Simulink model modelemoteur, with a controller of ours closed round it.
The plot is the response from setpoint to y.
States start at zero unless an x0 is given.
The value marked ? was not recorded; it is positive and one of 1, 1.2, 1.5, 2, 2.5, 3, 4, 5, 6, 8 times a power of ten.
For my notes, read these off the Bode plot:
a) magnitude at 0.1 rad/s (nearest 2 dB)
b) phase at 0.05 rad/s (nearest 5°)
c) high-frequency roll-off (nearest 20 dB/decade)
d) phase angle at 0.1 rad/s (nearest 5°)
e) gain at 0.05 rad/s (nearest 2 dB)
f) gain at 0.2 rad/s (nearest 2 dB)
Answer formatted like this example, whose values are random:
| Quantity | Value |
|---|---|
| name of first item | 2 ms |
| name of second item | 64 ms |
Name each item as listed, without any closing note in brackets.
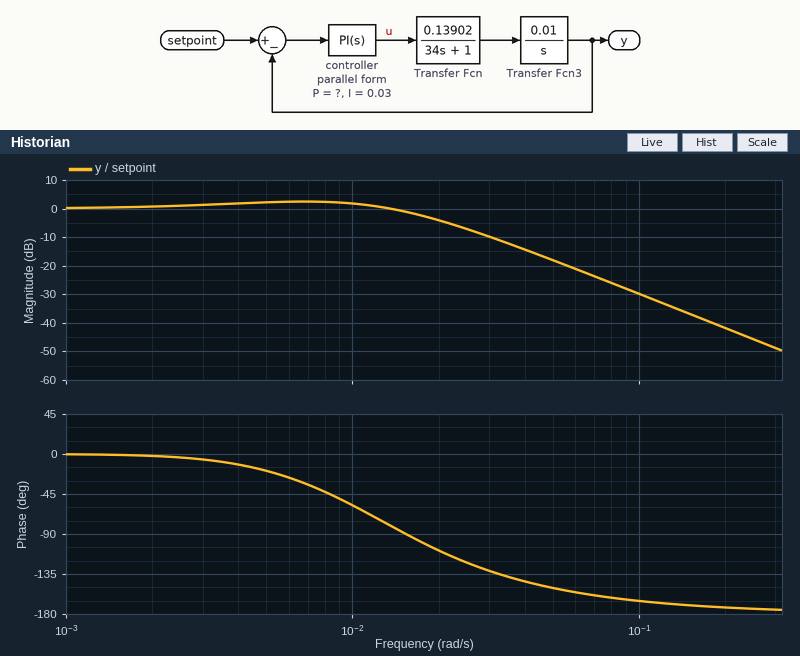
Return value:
| Quantity | Value |
|---|---|
| magnitude at 0.1 rad/s | -30 dB |
| phase at 0.05 rad/s | -150° |
| high-frequency roll-off | -40 dB/decade |
| phase angle at 0.1 rad/s | -165° |
| gain at 0.05 rad/s | -18 dB |
| gain at 0.2 rad/s | -42 dB |
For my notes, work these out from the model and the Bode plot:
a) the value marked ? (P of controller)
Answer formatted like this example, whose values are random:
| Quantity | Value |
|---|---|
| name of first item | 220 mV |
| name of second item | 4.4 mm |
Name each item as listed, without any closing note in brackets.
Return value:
| Quantity | Value |
|---|---|
| the value marked ? | 8 |
